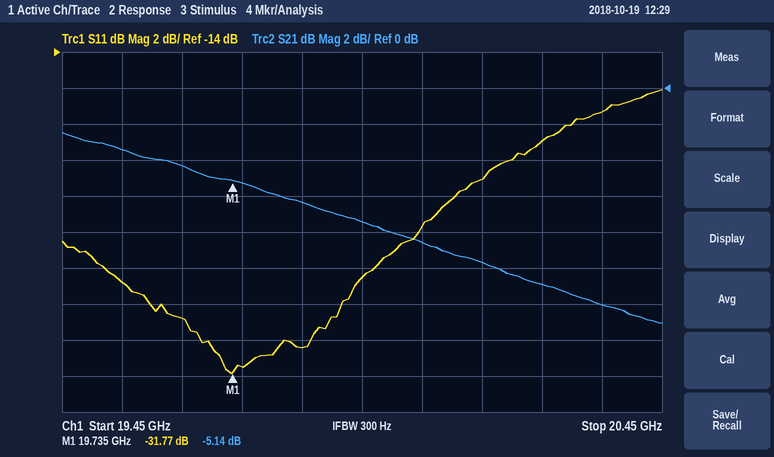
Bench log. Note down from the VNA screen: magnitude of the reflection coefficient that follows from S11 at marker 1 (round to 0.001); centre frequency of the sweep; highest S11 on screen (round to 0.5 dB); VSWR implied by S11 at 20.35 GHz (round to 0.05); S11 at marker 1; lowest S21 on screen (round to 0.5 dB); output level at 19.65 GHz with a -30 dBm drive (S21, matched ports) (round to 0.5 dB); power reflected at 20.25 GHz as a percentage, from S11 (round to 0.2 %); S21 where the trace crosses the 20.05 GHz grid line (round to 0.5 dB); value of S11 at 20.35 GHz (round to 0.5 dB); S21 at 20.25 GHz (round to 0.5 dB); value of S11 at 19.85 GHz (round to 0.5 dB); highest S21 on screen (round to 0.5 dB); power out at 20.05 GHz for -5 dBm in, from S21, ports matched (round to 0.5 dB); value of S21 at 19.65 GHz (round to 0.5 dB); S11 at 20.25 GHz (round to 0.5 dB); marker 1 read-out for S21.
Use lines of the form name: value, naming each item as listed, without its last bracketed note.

magnitude of the reflection coefficient that follows from S11 at marker 1: 0.026
centre frequency of the sweep: 19.95 GHz
highest S11 on screen: -16.0 dB
VSWR implied by S11 at 20.35 GHz: 1.30
S11 at marker 1: -31.77 dB
lowest S21 on screen: -13.0 dB
output level at 19.65 GHz with a -30 dBm drive (S21, matched ports): -34.5 dBm
power reflected at 20.25 GHz as a percentage, from S11: 1.2 %
S21 where the trace crosses the 20.05 GHz grid line: -8.5 dB
value of S11 at 20.35 GHz: -17.5 dB
S21 at 20.25 GHz: -11.0 dB
value of S11 at 19.85 GHz: -30.5 dB
highest S21 on screen: -2.5 dB
power out at 20.05 GHz for -5 dBm in, from S21, ports matched: -13.5 dBm
value of S21 at 19.65 GHz: -4.5 dB
S11 at 20.25 GHz: -19.0 dB
marker 1 read-out for S21: -5.14 dB
